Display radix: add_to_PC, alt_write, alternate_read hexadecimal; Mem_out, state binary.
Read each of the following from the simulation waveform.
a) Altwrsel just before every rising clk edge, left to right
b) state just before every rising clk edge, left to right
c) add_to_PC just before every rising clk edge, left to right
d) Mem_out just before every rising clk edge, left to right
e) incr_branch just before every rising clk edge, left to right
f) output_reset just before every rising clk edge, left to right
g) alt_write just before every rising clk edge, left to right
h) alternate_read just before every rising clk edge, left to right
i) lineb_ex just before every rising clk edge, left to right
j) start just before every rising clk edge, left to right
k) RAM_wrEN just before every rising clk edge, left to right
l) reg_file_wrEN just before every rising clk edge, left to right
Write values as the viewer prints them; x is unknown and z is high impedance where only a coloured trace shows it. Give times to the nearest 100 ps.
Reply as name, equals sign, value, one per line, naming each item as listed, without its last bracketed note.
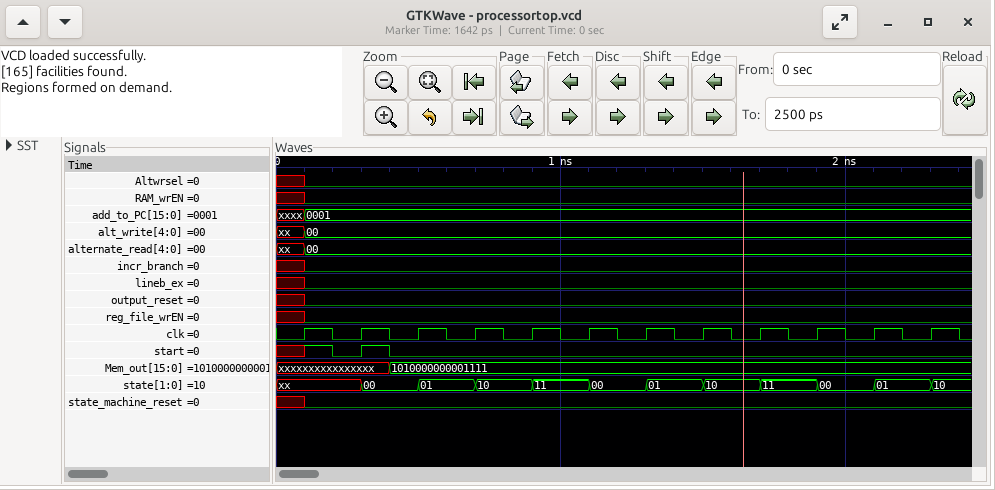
Altwrsel just before every rising clk edge, left to right = x 0 0 0 0 0 0 0 0 0 0 0
state just before every rising clk edge, left to right = xx, xx, 00, 01, 10, 11, 00, 01, 10, 11, 00, 01
add_to_PC just before every rising clk edge, left to right = xxxx, 0001, 0001, 0001, 0001, 0001, 0001, 0001, 0001, 0001, 0001, 0001
Mem_out just before every rising clk edge, left to right = xxxxxxxxxxxxxxxx, xxxxxxxxxxxxxxxx, 1010000000001111, 1010000000001111, 1010000000001111, 1010000000001111, 1010000000001111, 1010000000001111, 1010000000001111, 1010000000001111, 1010000000001111, 1010000000001111
incr_branch just before every rising clk edge, left to right = x 0 0 0 0 0 0 0 0 0 0 0
output_reset just before every rising clk edge, left to right = x 0 0 0 0 0 0 0 0 0 0 0
alt_write just before every rising clk edge, left to right = xx, 00, 00, 00, 00, 00, 00, 00, 00, 00, 00, 00
alternate_read just before every rising clk edge, left to right = xx, 00, 00, 00, 00, 00, 00, 00, 00, 00, 00, 00
lineb_ex just before every rising clk edge, left to right = x 0 0 0 0 0 0 0 0 0 0 0
start just before every rising clk edge, left to right = x 0 0 0 0 0 0 0 0 0 0 0
RAM_wrEN just before every rising clk edge, left to right = x 0 0 0 0 0 0 0 0 0 0 0
reg_file_wrEN just before every rising clk edge, left to right = x 0 0 0 0 0 0 0 0 0 0 0
